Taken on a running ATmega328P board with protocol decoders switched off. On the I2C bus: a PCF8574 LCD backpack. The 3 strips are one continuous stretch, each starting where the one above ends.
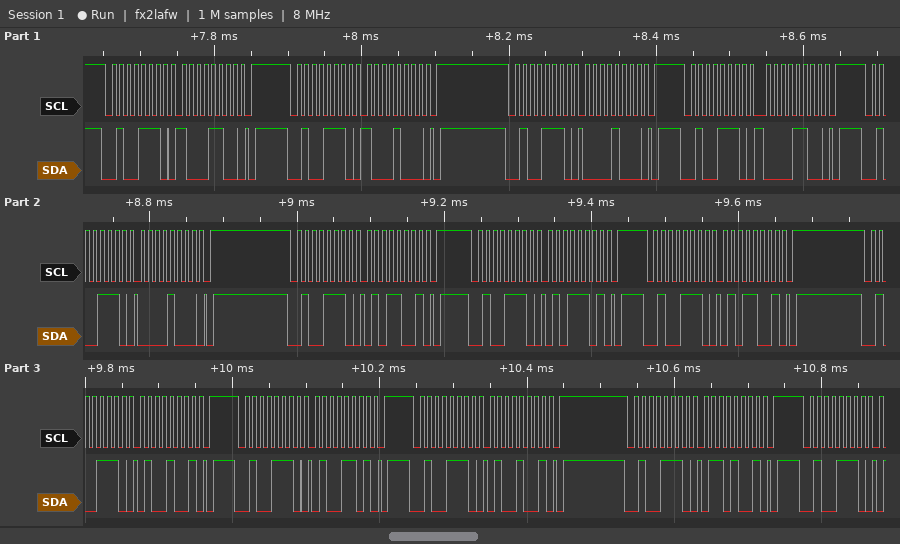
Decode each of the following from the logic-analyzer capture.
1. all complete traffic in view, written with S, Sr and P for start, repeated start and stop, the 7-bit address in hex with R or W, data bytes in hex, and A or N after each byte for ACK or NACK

S 27W A 8C A P S 27W A 88 A P S 27W A 08 A P S 27W A 0C A P S 27W A 08 A P S 27W A 59 A P S 27W A 5D A P S 27W A 59 A P S 27W A 49 A P S 27W A 4D A P S 27W A 49 A P S 27W A 69 A P S 27W A
